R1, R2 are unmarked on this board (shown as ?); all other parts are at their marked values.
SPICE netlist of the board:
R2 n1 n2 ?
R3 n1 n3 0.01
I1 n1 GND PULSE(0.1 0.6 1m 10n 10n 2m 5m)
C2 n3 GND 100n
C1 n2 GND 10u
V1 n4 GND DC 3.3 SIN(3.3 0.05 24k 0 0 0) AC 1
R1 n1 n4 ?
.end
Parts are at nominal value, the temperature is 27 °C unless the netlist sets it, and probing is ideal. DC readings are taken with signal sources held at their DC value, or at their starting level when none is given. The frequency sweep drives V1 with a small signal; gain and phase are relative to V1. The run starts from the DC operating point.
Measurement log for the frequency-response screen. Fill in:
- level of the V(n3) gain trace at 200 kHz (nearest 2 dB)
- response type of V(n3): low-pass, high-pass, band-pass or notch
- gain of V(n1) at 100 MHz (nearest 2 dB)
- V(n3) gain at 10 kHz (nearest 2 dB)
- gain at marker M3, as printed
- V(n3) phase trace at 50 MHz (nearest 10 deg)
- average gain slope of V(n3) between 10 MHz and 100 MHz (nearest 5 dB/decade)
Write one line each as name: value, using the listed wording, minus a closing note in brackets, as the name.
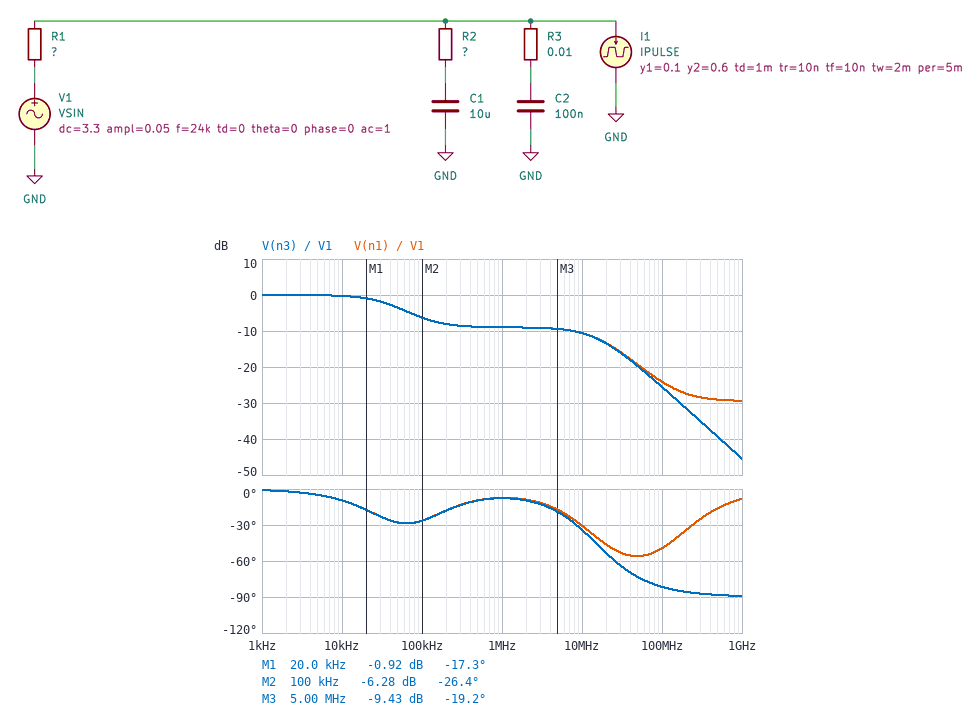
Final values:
level of the V(n3) gain trace at 200 kHz: -8 dB
response type of V(n3): low-pass, high-pass, band-pass or notch: low-pass
gain of V(n1) at 100 MHz: -24 dB
V(n3) gain at 10 kHz: 0 dB
gain at marker M3, as printed: -9.43 dB
V(n3) phase trace at 50 MHz: -70 deg
average gain slope of V(n3) between 10 MHz and 100 MHz: -15 dB/decade
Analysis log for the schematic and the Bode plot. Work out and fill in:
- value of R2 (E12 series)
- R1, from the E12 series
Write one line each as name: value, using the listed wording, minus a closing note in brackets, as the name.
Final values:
value of R2: 0.15 Ω
R1, from the E12 series: 0.27 Ω
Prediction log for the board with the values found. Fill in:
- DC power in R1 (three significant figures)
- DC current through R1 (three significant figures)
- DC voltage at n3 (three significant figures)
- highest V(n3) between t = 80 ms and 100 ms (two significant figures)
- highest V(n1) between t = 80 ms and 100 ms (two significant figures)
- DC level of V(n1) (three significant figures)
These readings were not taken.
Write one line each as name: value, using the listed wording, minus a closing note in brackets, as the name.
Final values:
DC power in R1: 2.70 mW
DC current through R1: 100 mA
DC voltage at n3: 3.27 V
highest V(n3) between t = 80 ms and 100 ms: 3.3 V
highest V(n1) between t = 80 ms and 100 ms: 3.3 V
DC level of V(n1): 3.27 V
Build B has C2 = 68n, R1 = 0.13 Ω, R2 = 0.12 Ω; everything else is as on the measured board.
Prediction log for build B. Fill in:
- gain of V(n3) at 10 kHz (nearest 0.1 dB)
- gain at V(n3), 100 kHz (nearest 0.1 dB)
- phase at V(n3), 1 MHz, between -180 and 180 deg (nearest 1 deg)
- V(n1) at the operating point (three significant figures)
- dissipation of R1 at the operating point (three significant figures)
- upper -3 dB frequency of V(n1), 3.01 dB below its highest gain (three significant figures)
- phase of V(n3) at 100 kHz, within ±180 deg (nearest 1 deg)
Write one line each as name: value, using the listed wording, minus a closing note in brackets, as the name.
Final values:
gain of V(n3) at 10 kHz: -0.1 dB
gain at V(n3), 100 kHz: -3.5 dB
phase at V(n3), 1 MHz, between -180 and 180 deg: -6 deg
V(n1) at the operating point: 3.29 V
dissipation of R1 at the operating point: 1.30 mW
upper -3 dB frequency of V(n1), 3.01 dB below its highest gain: 86.4 kHz
phase of V(n3) at 100 kHz, within ±180 deg: -21 deg
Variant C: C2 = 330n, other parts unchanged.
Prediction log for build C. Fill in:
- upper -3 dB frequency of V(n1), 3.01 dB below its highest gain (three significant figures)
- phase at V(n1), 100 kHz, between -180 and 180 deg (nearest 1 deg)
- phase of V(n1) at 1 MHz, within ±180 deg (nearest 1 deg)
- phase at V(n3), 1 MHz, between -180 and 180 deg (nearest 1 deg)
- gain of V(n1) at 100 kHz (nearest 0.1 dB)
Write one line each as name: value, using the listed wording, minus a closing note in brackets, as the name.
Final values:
upper -3 dB frequency of V(n1), 3.01 dB below its highest gain: 43.1 kHz
phase at V(n1), 100 kHz, between -180 and 180 deg: -27 deg
phase of V(n1) at 1 MHz, within ±180 deg: -15 deg
phase at V(n3), 1 MHz, between -180 and 180 deg: -16 deg
gain of V(n1) at 100 kHz: -6.4 dB
